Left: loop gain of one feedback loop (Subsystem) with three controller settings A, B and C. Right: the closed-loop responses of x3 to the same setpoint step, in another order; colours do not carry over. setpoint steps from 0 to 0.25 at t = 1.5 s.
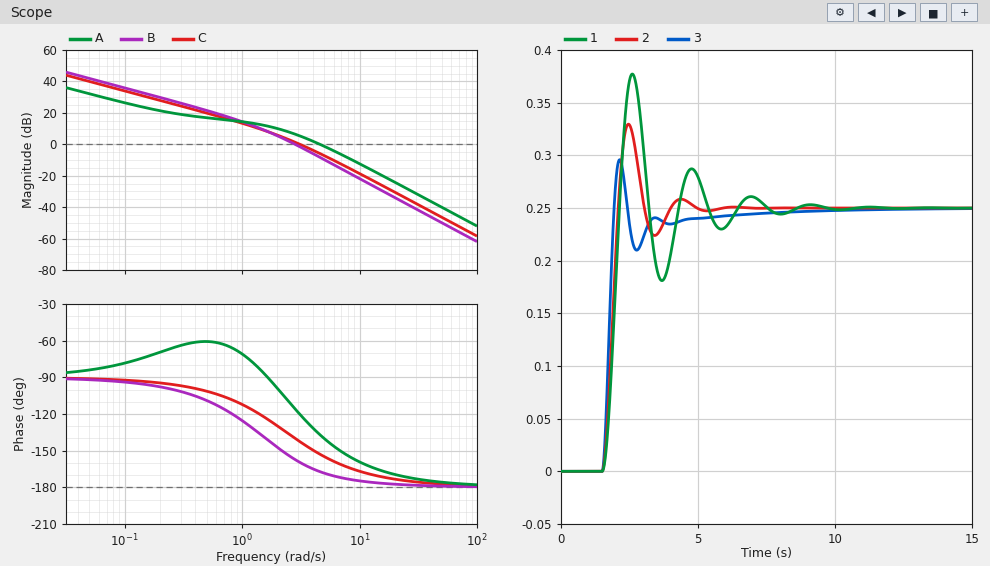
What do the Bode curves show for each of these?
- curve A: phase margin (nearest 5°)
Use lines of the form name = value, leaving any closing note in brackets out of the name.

curve A: phase margin = 45°
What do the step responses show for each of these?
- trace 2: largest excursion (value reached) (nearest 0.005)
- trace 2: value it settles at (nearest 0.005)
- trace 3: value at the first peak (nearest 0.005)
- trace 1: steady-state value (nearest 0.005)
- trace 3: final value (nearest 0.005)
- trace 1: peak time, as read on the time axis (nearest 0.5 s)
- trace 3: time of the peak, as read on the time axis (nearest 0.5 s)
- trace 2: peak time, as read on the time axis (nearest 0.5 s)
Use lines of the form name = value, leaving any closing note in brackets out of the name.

trace 2: largest excursion (value reached) = 0.330
trace 2: value it settles at = 0.250
trace 3: value at the first peak = 0.295
trace 1: steady-state value = 0.250
trace 3: final value = 0.250
trace 1: peak time, as read on the time axis = 2.5 s
trace 3: time of the peak, as read on the time axis = 2.0 s
trace 2: peak time, as read on the time axis = 2.5 s
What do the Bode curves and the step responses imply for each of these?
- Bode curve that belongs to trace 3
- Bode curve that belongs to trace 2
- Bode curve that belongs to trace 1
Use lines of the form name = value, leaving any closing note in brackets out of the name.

Bode curve that belongs to trace 3 = A
Bode curve that belongs to trace 2 = C
Bode curve that belongs to trace 1 = B
